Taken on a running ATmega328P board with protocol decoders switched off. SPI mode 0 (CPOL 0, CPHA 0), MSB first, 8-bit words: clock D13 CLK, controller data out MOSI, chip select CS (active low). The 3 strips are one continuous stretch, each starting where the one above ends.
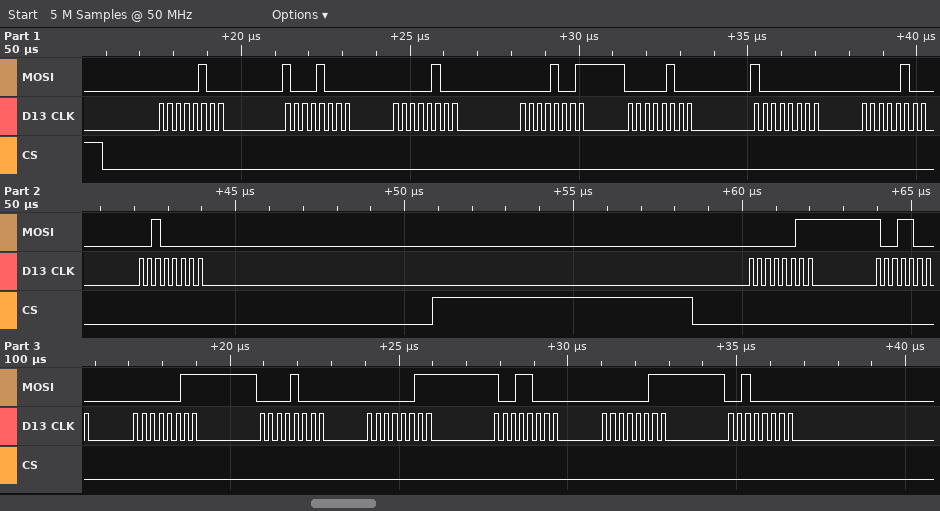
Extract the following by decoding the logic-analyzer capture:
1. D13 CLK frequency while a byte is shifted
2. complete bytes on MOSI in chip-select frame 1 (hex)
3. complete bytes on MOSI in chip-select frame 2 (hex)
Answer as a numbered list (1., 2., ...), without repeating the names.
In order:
1. 4 MHz
2. 04 88 04 09 04 80 04 20
3. 03 98 03 08 03 98 03 20
